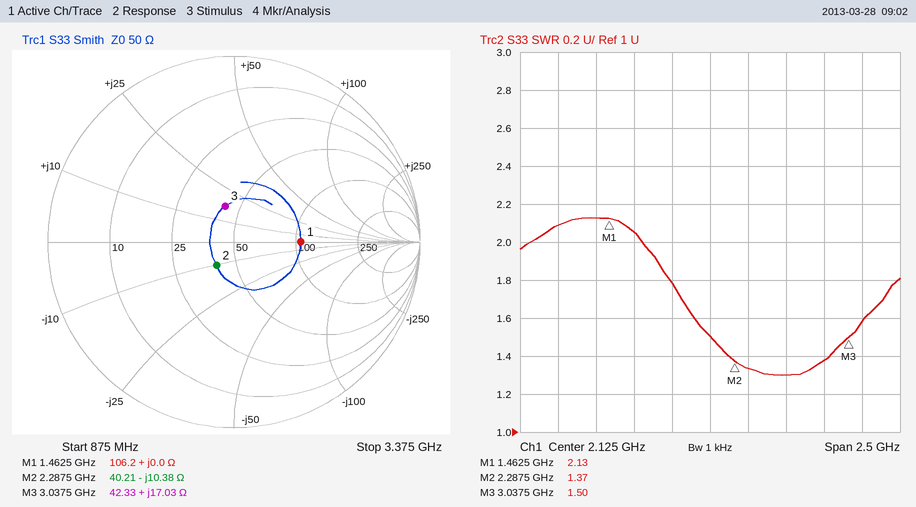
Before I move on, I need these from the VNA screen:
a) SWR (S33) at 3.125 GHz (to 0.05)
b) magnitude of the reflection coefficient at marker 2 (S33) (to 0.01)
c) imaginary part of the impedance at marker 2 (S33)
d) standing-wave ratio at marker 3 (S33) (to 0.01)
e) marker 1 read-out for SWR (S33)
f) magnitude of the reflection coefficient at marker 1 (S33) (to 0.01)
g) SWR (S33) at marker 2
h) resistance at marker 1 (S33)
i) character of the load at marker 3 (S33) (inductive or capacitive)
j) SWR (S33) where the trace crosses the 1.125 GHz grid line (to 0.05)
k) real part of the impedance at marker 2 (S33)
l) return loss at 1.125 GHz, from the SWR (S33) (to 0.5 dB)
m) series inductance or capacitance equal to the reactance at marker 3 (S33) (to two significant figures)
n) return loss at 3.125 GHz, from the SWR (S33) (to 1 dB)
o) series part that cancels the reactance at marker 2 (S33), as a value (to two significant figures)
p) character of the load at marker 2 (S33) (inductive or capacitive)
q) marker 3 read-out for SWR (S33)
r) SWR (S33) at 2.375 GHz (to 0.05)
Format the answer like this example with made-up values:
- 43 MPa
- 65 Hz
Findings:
- 1.60
- 0.16
- -10.38 Ω
- 1.50
- 2.13
- 0.36
- 1.37
- 106.2 Ω
- inductive
- 2.10
- 40.21 Ω
- 9.0 dB
- 890 pH
- 13 dB
- 720 pH
- capacitive
- 1.50
- 1.35
